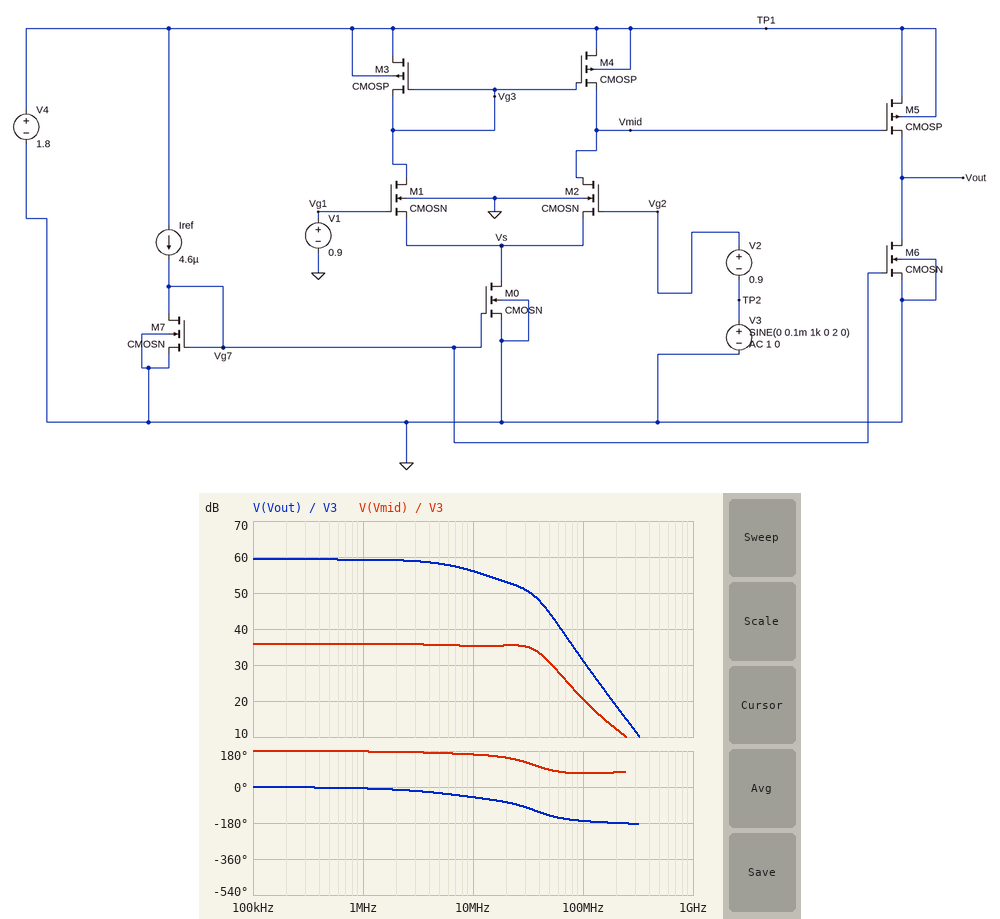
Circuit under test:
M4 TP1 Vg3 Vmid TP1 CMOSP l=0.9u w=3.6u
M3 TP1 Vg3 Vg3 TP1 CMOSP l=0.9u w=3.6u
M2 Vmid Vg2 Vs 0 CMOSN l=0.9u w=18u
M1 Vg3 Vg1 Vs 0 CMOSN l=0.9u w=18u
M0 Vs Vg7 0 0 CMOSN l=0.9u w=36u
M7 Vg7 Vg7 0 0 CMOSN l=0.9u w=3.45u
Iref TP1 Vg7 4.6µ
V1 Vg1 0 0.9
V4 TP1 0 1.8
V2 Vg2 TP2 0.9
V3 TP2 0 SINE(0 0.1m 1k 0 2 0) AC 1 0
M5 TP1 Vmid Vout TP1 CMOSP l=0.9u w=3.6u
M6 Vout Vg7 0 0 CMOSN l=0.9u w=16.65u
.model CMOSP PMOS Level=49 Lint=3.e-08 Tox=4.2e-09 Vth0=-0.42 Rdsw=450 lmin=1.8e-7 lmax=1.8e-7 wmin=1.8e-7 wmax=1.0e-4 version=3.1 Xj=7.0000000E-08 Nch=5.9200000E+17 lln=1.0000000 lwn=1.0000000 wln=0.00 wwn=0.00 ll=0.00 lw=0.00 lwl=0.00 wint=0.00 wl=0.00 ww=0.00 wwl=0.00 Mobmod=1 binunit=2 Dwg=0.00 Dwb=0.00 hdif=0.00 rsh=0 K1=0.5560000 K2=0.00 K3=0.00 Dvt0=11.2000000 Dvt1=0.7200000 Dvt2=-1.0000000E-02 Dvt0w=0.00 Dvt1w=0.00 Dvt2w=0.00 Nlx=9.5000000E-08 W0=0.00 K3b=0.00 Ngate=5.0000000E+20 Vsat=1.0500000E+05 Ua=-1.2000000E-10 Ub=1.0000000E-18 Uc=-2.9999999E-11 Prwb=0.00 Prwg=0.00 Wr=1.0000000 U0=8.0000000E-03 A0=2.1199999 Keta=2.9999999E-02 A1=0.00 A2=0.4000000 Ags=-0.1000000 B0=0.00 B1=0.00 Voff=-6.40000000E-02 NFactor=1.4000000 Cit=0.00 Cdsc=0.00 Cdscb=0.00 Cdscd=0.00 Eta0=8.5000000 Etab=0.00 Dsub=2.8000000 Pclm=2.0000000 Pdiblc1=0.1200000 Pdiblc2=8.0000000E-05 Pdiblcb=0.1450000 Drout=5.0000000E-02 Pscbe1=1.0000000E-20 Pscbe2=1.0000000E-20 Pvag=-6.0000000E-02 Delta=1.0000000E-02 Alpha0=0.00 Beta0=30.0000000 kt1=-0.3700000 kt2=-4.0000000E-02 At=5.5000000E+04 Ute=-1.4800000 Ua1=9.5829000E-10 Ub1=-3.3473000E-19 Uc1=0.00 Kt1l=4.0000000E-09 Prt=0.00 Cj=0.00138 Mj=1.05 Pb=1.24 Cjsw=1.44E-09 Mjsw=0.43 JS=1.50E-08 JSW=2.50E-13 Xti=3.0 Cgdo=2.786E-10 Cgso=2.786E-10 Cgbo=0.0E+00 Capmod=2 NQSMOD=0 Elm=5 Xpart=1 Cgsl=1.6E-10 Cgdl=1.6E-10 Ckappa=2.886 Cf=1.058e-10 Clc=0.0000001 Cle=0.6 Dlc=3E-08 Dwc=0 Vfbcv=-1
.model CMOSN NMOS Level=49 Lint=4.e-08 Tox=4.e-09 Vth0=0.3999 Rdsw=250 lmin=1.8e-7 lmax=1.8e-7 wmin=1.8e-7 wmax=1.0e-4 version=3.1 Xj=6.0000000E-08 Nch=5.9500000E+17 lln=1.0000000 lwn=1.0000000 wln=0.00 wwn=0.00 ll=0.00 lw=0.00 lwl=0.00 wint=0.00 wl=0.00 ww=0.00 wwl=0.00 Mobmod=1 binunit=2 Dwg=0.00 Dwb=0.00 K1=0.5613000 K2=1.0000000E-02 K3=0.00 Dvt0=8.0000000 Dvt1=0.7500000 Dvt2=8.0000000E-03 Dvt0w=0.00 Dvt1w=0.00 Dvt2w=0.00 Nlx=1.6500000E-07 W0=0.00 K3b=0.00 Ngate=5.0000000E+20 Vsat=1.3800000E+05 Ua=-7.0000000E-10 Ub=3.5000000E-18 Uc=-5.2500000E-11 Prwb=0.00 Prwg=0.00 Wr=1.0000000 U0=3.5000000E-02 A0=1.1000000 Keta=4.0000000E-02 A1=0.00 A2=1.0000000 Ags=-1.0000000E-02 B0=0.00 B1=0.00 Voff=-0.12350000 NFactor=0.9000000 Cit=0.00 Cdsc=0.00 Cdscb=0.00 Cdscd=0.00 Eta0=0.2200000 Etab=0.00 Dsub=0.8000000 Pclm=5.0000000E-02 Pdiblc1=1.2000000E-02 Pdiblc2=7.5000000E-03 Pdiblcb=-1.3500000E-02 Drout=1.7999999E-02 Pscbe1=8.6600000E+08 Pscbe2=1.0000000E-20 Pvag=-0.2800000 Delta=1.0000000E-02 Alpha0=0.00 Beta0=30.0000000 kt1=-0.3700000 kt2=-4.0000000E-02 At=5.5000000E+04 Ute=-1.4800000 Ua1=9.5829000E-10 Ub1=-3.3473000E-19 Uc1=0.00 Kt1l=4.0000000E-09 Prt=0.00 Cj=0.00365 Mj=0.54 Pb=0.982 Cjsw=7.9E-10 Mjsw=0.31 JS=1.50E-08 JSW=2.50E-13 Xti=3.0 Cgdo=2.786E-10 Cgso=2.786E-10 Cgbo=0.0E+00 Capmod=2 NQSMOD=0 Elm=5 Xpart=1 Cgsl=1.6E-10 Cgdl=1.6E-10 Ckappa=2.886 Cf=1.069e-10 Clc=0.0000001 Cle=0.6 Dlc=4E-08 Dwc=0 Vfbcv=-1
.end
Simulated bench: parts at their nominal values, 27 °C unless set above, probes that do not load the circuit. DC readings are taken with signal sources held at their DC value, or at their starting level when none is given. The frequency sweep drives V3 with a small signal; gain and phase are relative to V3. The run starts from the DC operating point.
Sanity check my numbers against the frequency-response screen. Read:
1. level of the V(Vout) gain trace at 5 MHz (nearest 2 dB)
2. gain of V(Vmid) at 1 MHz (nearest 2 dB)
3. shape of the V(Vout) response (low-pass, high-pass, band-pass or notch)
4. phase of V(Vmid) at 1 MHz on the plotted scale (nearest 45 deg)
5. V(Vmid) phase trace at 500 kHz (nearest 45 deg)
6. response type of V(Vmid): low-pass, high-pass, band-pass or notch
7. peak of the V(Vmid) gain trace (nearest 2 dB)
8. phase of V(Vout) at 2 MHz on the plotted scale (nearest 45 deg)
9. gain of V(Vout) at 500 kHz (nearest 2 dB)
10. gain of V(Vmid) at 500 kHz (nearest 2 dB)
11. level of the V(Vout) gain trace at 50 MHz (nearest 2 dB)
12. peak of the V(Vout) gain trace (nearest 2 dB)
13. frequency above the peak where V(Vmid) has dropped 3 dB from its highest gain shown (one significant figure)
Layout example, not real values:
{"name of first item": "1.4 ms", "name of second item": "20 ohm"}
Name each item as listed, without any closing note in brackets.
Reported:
{"level of the V(Vout) gain trace at 5 MHz": "58 dB", "gain of V(Vmid) at 1 MHz": "36 dB", "shape of the V(Vout) response": "low-pass", "phase of V(Vmid) at 1 MHz on the plotted scale": "180 deg", "V(Vmid) phase trace at 500 kHz": "180 deg", "response type of V(Vmid): low-pass, high-pass, band-pass or notch": "low-pass", "peak of the V(Vmid) gain trace": "36 dB", "phase of V(Vout) at 2 MHz on the plotted scale": "0 deg", "gain of V(Vout) at 500 kHz": "60 dB", "gain of V(Vmid) at 500 kHz": "36 dB", "level of the V(Vout) gain trace at 50 MHz": "44 dB", "peak of the V(Vout) gain trace": "60 dB", "frequency above the peak where V(Vmid) has dropped 3 dB from its highest gain shown": "40 MHz"}
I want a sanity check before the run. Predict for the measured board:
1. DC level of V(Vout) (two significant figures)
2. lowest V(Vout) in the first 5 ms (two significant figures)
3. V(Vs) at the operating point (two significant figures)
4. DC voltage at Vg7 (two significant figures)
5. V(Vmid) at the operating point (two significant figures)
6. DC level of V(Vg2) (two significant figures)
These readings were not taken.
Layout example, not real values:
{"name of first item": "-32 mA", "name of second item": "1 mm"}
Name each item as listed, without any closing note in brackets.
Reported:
{"DC level of V(Vout)": "870 mV", "lowest V(Vout) in the first 5 ms": "780 mV", "V(Vs) at the operating point": "300 mV", "DC voltage at Vg7": "510 mV", "V(Vmid) at the operating point": "860 mV", "DC level of V(Vg2)": "900 mV"}
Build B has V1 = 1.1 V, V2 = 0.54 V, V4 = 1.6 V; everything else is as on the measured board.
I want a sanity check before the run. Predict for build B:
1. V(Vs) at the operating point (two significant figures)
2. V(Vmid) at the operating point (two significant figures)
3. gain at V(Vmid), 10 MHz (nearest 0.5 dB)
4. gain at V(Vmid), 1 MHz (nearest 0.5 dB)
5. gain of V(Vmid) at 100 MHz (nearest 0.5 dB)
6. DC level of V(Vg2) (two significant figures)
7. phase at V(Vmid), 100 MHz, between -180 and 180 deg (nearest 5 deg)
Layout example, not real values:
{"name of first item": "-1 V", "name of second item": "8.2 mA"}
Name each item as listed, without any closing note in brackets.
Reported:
{"V(Vs) at the operating point": "370 mV", "V(Vmid) at the operating point": "1.6 V", "gain at V(Vmid), 10 MHz": "-50.0 dB", "gain at V(Vmid), 1 MHz": "-70.0 dB", "gain of V(Vmid) at 100 MHz": "-30.0 dB", "DC level of V(Vg2)": "540 mV", "phase at V(Vmid), 100 MHz, between -180 and 180 deg": "80 deg"}
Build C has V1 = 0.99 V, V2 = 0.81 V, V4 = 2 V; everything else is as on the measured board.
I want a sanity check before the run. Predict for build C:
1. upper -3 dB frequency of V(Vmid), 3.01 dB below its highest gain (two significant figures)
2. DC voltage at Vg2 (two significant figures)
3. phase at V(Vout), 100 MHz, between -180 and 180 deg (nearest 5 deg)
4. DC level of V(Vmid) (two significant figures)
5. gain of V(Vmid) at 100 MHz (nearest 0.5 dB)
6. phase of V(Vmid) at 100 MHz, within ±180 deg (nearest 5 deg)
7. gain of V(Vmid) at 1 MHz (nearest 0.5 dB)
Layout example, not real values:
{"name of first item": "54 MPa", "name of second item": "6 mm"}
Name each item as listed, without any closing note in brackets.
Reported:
{"upper -3 dB frequency of V(Vmid), 3.01 dB below its highest gain": "520 MHz", "DC voltage at Vg2": "810 mV", "phase at V(Vout), 100 MHz, between -180 and 180 deg": "-150 deg", "DC level of V(Vmid)": "2.0 V", "gain of V(Vmid) at 100 MHz": "-12.0 dB", "phase of V(Vmid) at 100 MHz, within ±180 deg": "155 deg", "gain of V(Vmid) at 1 MHz": "-11.5 dB"}
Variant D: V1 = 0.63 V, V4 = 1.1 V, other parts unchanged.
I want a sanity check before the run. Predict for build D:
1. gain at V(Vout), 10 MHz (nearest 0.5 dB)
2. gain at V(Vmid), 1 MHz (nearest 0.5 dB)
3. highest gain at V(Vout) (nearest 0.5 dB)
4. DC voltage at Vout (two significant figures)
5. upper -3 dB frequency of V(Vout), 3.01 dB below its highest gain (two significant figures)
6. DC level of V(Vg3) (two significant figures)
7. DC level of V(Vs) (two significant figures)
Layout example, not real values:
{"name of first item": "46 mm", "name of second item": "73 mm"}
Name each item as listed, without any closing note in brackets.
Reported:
{"gain at V(Vout), 10 MHz": "-25.0 dB", "gain at V(Vmid), 1 MHz": "-29.5 dB", "highest gain at V(Vout)": "-10.0 dB", "DC voltage at Vout": "830 mV", "upper -3 dB frequency of V(Vout), 3.01 dB below its highest gain": "600 MHz", "DC level of V(Vg3)": "190 mV", "DC level of V(Vs)": "92 mV"}
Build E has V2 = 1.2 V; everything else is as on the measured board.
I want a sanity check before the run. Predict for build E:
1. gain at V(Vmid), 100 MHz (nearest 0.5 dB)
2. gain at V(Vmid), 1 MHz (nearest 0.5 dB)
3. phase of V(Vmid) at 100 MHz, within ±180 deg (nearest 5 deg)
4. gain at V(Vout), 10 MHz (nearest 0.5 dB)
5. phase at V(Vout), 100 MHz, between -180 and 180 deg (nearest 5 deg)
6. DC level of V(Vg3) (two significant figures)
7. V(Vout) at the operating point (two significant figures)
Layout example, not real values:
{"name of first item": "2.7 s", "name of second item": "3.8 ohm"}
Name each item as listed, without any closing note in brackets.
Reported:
{"gain at V(Vmid), 100 MHz": "-17.5 dB", "gain at V(Vmid), 1 MHz": "-29.5 dB", "phase of V(Vmid) at 100 MHz, within ±180 deg": "105 deg", "gain at V(Vout), 10 MHz": "-47.0 dB", "phase at V(Vout), 100 MHz, between -180 and 180 deg": "-100 deg", "DC level of V(Vg3)": "870 mV", "V(Vout) at the operating point": "1.7 V"}
